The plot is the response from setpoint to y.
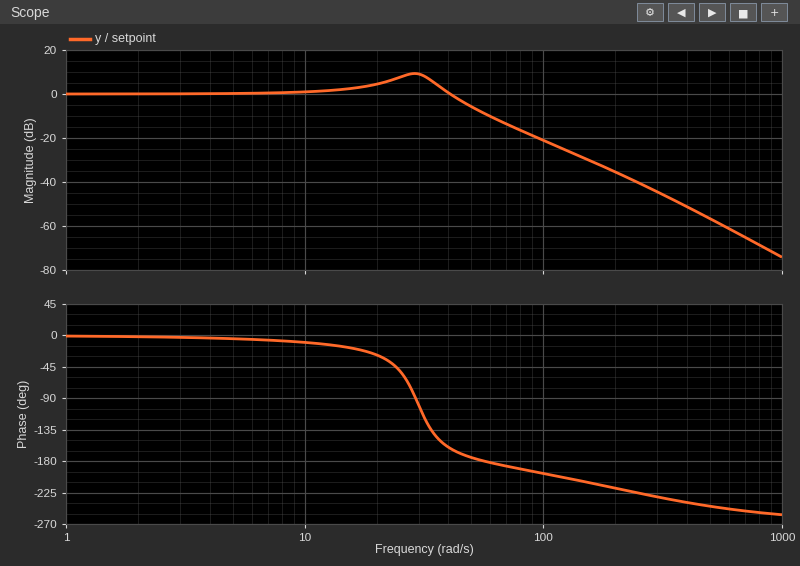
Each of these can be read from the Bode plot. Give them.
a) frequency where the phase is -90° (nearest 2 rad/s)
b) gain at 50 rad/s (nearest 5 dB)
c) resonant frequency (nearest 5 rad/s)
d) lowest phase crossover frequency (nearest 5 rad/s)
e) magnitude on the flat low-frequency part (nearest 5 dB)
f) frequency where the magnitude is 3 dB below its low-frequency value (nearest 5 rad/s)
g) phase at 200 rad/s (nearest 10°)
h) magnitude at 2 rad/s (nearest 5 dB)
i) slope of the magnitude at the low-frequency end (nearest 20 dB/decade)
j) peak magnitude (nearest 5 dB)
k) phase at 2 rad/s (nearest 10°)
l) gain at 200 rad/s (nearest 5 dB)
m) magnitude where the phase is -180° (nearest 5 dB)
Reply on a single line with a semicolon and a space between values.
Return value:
30 rad/s; -5 dB; 30 rad/s; 55 rad/s; 0 dB; 45 rad/s; -220°; 0 dB; 0 dB/decade; 10 dB; 0°; -35 dB; -10 dB
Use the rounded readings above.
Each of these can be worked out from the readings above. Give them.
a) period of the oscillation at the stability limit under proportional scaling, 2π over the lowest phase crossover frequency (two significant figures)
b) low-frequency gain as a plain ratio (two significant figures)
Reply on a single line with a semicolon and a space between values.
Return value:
0.11 s; 1.0
